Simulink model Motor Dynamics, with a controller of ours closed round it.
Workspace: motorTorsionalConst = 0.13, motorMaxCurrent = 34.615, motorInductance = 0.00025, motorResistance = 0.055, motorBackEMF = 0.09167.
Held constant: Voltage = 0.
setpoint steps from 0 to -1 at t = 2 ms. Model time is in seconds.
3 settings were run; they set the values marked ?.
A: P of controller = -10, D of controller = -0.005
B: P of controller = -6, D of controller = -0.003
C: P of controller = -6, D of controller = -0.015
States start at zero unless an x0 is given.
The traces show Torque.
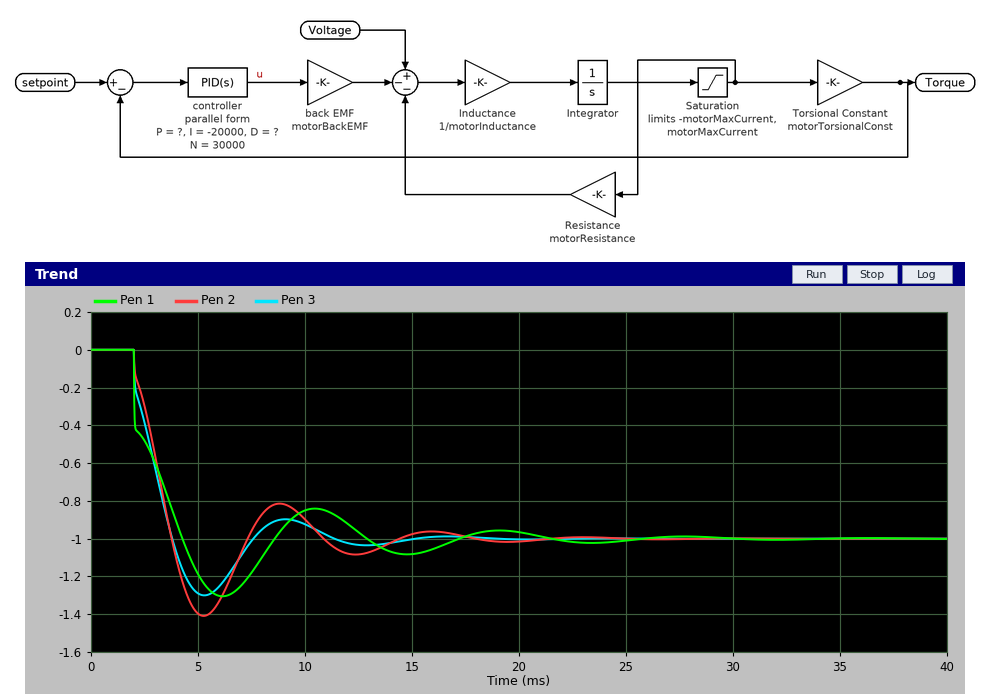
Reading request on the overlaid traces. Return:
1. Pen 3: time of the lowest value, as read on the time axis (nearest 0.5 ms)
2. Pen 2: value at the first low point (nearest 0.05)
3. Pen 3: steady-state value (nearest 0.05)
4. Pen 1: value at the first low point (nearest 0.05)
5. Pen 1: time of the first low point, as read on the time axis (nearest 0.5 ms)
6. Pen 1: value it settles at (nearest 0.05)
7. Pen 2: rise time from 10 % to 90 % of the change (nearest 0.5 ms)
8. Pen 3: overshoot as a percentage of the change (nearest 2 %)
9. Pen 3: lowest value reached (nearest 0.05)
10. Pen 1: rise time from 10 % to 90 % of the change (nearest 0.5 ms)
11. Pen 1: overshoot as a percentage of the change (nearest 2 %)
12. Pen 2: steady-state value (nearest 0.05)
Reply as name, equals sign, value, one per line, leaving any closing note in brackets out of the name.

Pen 3: time of the lowest value, as read on the time axis = 5.5 ms
Pen 2: value at the first low point = -1.40
Pen 3: steady-state value = -1.00
Pen 1: value at the first low point = -1.30
Pen 1: time of the first low point, as read on the time axis = 6.0 ms
Pen 1: value it settles at = -1.00
Pen 2: rise time from 10 % to 90 % of the change = 1.5 ms
Pen 3: overshoot as a percentage of the change = 30 %
Pen 3: lowest value reached = -1.30
Pen 1: rise time from 10 % to 90 % of the change = 2.0 ms
Pen 1: overshoot as a percentage of the change = 30 %
Pen 2: steady-state value = -1.00
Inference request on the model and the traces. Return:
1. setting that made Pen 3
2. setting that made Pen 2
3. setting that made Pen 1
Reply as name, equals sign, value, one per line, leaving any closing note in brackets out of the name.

setting that made Pen 3 = A
setting that made Pen 2 = B
setting that made Pen 1 = C
